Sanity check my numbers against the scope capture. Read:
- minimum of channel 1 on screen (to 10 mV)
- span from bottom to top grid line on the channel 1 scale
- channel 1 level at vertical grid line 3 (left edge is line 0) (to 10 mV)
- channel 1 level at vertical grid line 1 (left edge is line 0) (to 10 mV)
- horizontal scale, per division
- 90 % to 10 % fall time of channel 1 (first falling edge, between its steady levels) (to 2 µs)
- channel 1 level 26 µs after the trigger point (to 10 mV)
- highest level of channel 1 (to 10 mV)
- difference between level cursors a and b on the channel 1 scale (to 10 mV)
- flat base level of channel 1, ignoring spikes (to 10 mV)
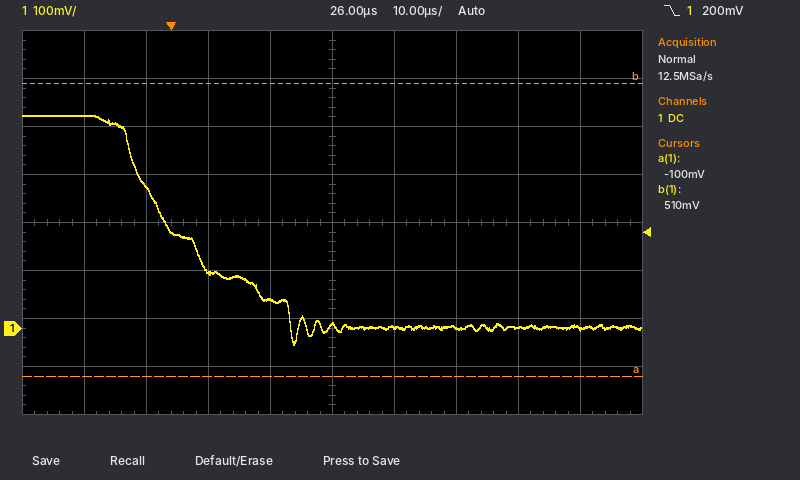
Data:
-30 mV
800 mV
120 mV
440 mV
10 µs
26 µs
10 mV
440 mV
610 mV
0 mV
